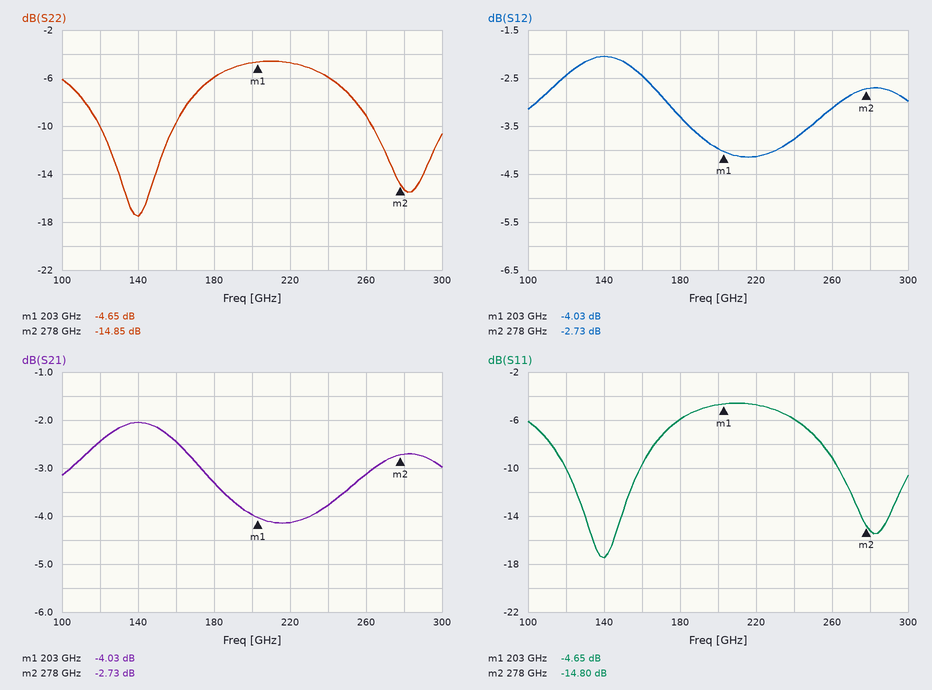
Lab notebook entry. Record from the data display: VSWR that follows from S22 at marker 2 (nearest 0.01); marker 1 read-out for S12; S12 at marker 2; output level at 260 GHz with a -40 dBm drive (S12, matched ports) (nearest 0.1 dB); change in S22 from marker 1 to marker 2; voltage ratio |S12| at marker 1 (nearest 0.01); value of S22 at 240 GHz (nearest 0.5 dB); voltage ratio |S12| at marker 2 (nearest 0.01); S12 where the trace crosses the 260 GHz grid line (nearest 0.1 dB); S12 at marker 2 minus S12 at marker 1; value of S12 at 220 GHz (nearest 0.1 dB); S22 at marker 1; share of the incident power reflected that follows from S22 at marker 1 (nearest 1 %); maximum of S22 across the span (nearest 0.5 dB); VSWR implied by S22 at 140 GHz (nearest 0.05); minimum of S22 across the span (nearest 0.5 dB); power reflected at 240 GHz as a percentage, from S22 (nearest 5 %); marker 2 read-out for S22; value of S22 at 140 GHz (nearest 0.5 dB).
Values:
1.44
-4.03 dB
-2.73 dB
-43.1 dBm
-10.20 dB
0.63
-6.0 dB
0.73
-3.1 dB
1.30 dB
-4.1 dB
-4.65 dB
34 %
-4.5 dB
1.30
-17.5 dB
25 %
-14.85 dB
-17.5 dB
